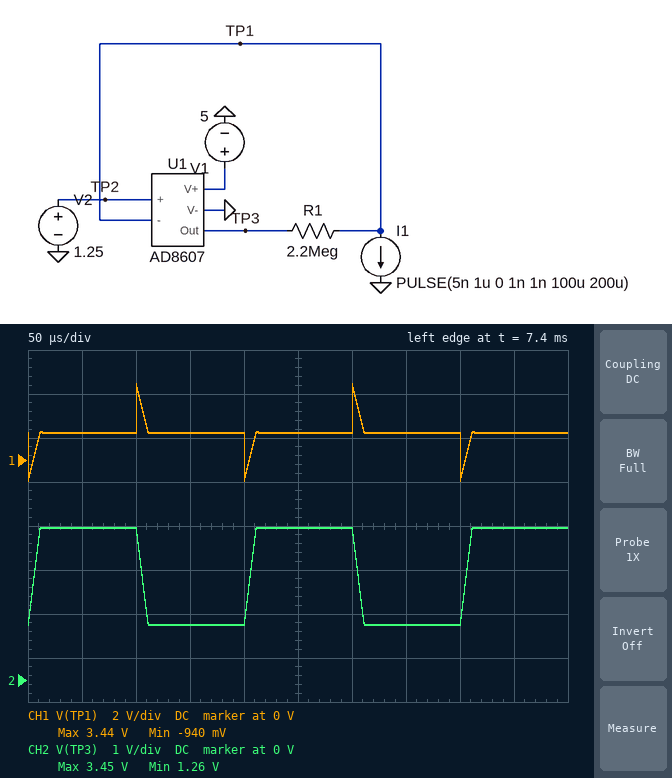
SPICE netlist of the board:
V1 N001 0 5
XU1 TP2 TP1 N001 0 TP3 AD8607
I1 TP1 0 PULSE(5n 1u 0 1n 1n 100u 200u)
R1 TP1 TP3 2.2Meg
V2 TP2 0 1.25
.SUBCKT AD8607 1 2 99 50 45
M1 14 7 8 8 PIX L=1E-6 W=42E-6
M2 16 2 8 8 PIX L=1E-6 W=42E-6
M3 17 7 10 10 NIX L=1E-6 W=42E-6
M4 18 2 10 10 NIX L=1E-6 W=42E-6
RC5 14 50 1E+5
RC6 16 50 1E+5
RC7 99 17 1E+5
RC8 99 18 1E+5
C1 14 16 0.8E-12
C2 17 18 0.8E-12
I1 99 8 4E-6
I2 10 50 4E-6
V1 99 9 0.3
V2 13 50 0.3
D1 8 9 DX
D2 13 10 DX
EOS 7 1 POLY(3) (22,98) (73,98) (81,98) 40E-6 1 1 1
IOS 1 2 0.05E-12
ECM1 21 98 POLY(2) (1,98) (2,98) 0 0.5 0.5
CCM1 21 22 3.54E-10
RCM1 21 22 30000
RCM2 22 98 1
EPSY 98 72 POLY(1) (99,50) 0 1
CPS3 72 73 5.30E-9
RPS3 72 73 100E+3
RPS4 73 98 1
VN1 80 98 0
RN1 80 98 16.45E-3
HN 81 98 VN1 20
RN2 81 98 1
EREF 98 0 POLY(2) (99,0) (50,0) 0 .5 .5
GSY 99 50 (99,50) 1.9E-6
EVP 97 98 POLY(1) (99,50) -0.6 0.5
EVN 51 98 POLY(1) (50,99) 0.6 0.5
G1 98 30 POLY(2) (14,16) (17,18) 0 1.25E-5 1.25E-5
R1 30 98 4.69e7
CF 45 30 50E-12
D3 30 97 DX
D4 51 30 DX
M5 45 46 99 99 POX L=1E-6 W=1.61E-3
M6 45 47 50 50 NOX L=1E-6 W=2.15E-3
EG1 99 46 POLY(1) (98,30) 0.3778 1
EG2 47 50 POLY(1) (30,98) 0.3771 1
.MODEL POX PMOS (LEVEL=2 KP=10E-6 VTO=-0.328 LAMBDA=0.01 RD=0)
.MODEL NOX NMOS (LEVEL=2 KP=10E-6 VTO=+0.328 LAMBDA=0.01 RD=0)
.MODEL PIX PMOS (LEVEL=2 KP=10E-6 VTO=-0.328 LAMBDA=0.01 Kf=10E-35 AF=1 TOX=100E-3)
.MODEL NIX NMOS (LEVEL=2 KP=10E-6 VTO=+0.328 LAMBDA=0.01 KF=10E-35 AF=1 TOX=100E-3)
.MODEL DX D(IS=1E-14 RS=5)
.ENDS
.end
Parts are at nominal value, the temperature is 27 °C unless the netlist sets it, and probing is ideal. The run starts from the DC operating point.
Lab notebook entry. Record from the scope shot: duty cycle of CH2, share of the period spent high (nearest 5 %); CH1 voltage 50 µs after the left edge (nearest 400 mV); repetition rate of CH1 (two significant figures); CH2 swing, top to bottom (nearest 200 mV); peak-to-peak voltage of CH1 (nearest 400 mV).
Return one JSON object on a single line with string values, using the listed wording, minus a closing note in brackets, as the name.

{"duty cycle of CH2, share of the period spent high": "50 %", "CH1 voltage 50 µs after the left edge": "1.2 V", "repetition rate of CH1": "5.0 kHz", "CH2 swing, top to bottom": "2.2 V", "peak-to-peak voltage of CH1": "4.4 V"}
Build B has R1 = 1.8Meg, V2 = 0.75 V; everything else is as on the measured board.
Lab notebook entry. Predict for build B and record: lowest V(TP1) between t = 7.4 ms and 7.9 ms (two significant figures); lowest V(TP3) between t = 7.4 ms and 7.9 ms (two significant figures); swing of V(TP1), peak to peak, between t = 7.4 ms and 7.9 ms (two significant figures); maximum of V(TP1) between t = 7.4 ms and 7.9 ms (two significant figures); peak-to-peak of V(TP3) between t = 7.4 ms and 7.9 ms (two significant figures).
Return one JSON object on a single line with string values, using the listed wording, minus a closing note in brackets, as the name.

{"lowest V(TP1) between t = 7.4 ms and 7.9 ms": "-1.0 V", "lowest V(TP3) between t = 7.4 ms and 7.9 ms": "760 mV", "swing of V(TP1), peak to peak, between t = 7.4 ms and 7.9 ms": "3.6 V", "maximum of V(TP1) between t = 7.4 ms and 7.9 ms": "2.5 V", "peak-to-peak of V(TP3) between t = 7.4 ms and 7.9 ms": "1.8 V"}
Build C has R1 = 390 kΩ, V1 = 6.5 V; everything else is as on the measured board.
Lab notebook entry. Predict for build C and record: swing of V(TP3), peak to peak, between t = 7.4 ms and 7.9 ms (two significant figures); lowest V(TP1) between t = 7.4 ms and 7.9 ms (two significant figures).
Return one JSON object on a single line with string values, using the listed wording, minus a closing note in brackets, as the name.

{"swing of V(TP3), peak to peak, between t = 7.4 ms and 7.9 ms": "390 mV", "lowest V(TP1) between t = 7.4 ms and 7.9 ms": "860 mV"}
